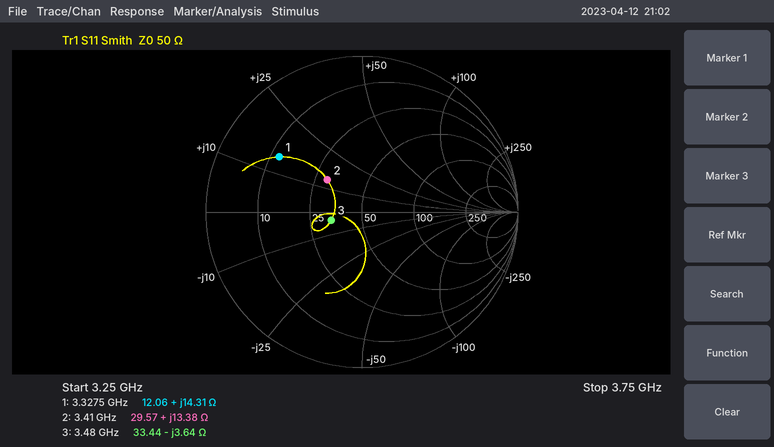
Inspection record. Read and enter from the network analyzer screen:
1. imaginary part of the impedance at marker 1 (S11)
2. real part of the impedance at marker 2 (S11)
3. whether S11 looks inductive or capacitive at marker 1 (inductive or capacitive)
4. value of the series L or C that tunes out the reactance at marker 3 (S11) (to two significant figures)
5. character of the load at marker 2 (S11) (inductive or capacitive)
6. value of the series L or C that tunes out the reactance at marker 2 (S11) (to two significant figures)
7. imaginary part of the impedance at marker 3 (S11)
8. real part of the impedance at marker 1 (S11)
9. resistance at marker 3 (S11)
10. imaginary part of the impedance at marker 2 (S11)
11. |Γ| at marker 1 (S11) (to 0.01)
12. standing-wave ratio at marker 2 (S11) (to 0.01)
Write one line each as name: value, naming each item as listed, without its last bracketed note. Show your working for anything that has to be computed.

imaginary part of the impedance at marker 1: +14.31 Ω
real part of the impedance at marker 2: 29.57 Ω
whether S11 looks inductive or capacitive at marker 1: inductive
value of the series L or C that tunes out the reactance at marker 3 (S11): L = 3.64 Ω/(2π × 3.48 GHz) ≈ 166 pH, so 170 pH to two significant figures
character of the load at marker 2 (S11): inductive
value of the series L or C that tunes out the reactance at marker 2 (S11): C = 1/(2π × 3.41 GHz × 13.38 Ω) ≈ 3.5 pF
imaginary part of the impedance at marker 3: -3.64 Ω
real part of the impedance at marker 1: 12.06 Ω
resistance at marker 3: 33.44 Ω
imaginary part of the impedance at marker 2: +13.38 Ω
|Γ| at marker 1 (S11): 0.64
standing-wave ratio at marker 2 (S11): 1.87
